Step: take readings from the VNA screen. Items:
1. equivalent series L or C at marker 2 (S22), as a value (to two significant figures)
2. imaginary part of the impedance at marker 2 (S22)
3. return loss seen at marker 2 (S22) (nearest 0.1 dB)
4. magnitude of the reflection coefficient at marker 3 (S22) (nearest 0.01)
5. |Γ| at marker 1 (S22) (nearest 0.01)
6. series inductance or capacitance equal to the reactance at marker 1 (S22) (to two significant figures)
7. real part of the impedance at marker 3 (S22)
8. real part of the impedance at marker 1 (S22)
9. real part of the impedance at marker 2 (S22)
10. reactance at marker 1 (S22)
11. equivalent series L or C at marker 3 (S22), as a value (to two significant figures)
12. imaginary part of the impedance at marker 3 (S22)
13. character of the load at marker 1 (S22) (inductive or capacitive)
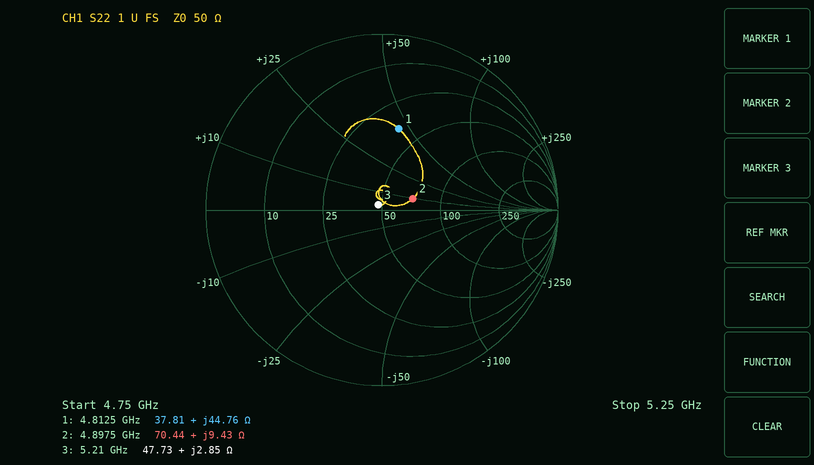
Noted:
310 pH
+9.43 Ω
14.6 dB
0.04
0.47
1.5 nH
47.73 Ω
37.81 Ω
70.44 Ω
+44.76 Ω
87 pH
+2.85 Ω
inductive
